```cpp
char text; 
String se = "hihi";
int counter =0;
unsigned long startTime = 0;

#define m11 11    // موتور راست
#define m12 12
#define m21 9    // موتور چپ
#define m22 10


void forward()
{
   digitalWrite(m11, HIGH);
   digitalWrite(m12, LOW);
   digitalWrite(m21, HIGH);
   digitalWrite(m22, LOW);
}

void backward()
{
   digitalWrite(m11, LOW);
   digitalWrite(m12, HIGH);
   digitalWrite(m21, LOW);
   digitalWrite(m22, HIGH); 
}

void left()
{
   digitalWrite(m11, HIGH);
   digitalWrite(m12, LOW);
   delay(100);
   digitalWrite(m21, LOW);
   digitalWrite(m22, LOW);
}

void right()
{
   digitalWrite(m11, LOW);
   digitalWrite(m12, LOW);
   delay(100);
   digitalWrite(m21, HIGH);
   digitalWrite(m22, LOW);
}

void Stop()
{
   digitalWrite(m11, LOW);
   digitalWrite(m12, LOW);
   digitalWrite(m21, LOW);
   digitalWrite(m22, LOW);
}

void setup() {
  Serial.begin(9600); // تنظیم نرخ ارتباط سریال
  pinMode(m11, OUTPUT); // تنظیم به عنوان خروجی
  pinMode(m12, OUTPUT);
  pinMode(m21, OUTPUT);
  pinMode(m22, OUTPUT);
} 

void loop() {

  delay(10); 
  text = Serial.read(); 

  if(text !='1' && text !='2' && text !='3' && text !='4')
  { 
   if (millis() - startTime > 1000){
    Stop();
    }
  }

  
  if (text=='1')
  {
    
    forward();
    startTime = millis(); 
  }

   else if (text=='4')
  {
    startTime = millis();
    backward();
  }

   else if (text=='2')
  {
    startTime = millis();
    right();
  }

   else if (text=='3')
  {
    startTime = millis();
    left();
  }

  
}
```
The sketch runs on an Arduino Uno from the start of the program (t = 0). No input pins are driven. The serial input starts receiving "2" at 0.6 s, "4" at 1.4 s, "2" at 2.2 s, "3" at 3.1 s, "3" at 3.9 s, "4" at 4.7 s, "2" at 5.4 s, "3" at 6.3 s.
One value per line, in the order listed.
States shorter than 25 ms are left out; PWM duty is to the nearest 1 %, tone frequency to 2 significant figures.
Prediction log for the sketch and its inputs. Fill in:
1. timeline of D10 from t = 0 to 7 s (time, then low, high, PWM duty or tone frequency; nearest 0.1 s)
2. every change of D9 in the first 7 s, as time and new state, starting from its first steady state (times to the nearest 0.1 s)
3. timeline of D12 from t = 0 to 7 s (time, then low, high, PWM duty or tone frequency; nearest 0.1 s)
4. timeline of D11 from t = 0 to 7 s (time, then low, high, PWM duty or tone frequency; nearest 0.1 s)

0 s low; 1.4 s high; 2.3 s low; 4.7 s high; 5.5 s low
0 s low; 0.7 s high; 1.4 s low; 2.3 s high; 3.2 s low; 5.5 s high; 6.4 s low
0 s low; 1.4 s high; 2.2 s low; 4.7 s high; 5.4 s low
0 s low; 3.1 s high; 4.7 s low; 6.3 s high
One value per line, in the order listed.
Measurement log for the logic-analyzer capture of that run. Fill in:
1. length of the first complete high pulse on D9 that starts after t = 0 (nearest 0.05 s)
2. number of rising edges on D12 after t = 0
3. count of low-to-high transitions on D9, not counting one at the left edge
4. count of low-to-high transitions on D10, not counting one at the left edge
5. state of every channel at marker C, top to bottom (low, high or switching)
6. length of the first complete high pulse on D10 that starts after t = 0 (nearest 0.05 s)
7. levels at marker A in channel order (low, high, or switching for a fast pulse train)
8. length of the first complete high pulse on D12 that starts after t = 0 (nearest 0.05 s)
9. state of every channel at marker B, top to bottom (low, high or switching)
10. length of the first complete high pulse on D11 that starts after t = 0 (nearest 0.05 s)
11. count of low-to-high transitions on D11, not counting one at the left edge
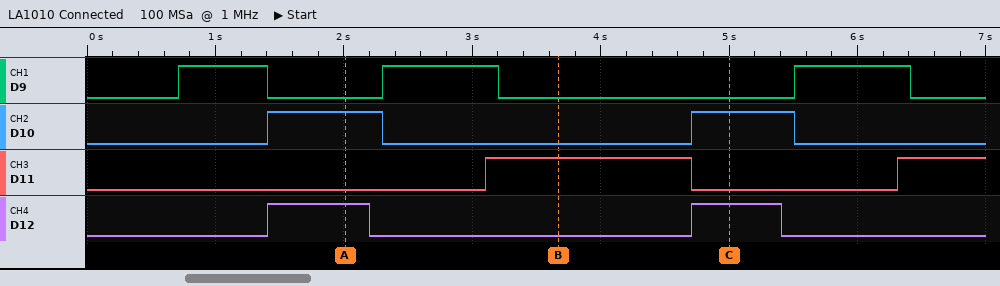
0.70 s
2
3
2
D9 low, D10 high, D11 low, D12 high
0.90 s
D9 low, D10 high, D11 low, D12 high
0.80 s
D9 low, D10 low, D11 high, D12 low
1.60 s
2
